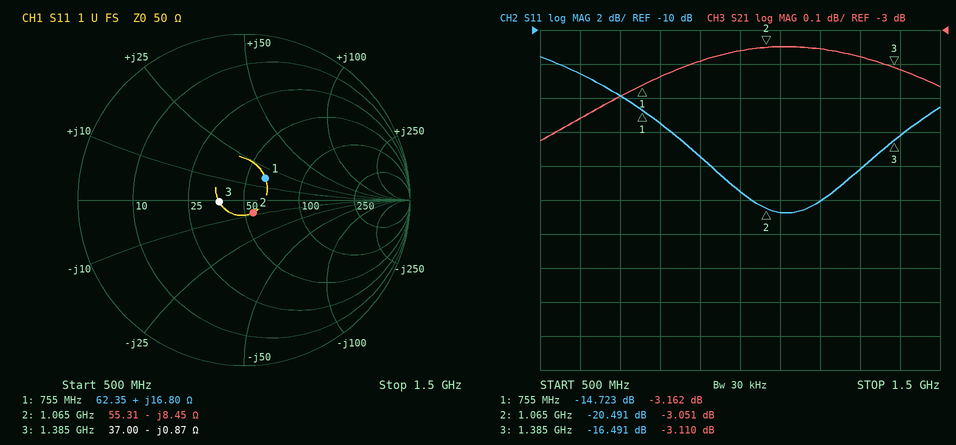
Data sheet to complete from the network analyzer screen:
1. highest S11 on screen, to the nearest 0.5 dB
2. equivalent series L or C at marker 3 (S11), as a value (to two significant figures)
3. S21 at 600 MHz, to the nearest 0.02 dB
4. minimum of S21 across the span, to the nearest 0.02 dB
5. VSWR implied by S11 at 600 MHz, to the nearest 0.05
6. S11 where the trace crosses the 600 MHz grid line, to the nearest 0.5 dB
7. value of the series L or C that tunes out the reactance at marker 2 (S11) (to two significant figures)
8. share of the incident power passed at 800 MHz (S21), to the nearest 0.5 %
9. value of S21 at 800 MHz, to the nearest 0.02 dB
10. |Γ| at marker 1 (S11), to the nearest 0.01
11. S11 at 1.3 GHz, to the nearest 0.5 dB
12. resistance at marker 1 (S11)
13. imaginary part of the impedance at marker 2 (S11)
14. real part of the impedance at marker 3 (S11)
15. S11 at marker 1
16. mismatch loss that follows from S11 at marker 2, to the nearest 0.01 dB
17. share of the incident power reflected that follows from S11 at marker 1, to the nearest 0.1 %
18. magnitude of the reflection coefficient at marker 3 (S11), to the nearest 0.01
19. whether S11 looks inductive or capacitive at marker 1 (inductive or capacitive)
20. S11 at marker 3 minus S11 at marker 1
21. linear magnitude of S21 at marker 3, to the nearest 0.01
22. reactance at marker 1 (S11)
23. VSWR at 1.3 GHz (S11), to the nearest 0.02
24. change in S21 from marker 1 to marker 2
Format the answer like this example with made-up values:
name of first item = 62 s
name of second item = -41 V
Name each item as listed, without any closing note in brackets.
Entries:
highest S11 on screen, to the nearest 0.5 dB = -11.5 dB
equivalent series L or C at marker 3 (S11), as a value = 130 pF
S21 at 600 MHz, to the nearest 0.02 dB = -3.26 dB
minimum of S21 across the span, to the nearest 0.02 dB = -3.32 dB
VSWR implied by S11 at 600 MHz, to the nearest 0.05 = 1.60
S11 where the trace crosses the 600 MHz grid line, to the nearest 0.5 dB = -12.5 dB
value of the series L or C that tunes out the reactance at marker 2 (S11) = 1.3 nH
share of the incident power passed at 800 MHz (S21), to the nearest 0.5 % = 48.5 %
value of S21 at 800 MHz, to the nearest 0.02 dB = -3.14 dB
|Γ| at marker 1 (S11), to the nearest 0.01 = 0.18
S11 at 1.3 GHz, to the nearest 0.5 dB = -18.0 dB
resistance at marker 1 = 62.35 Ω
imaginary part of the impedance at marker 2 = -8.45 Ω
real part of the impedance at marker 3 = 37.00 Ω
S11 at marker 1 = -14.723 dB
mismatch loss that follows from S11 at marker 2, to the nearest 0.01 dB = 0.04 dB
share of the incident power reflected that follows from S11 at marker 1, to the nearest 0.1 % = 3.4 %
magnitude of the reflection coefficient at marker 3 (S11), to the nearest 0.01 = 0.15
whether S11 looks inductive or capacitive at marker 1 = inductive
S11 at marker 3 minus S11 at marker 1 = -1.768 dB
linear magnitude of S21 at marker 3, to the nearest 0.01 = 0.70
reactance at marker 1 = +16.80 Ω
VSWR at 1.3 GHz (S11), to the nearest 0.02 = 1.28
change in S21 from marker 1 to marker 2 = 0.111 dB
